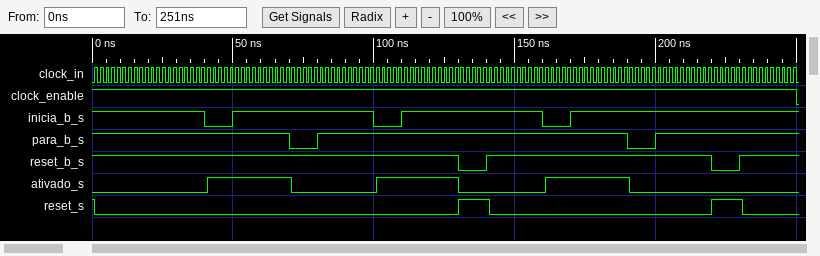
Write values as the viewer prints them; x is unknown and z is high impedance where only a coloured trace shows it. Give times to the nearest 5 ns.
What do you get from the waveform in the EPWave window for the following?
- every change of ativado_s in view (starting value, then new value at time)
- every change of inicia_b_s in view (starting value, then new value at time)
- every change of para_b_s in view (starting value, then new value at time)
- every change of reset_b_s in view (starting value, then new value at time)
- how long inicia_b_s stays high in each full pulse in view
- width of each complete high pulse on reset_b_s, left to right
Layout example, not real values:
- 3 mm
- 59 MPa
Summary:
- 0, 1 at 40 ns, 0 at 70 ns, 1 at 100 ns, 0 at 130 ns, 1 at 160 ns, 0 at 190 ns
- 1, 0 at 40 ns, 1 at 50 ns, 0 at 100 ns, 1 at 110 ns, 0 at 160 ns, 1 at 170 ns
- 1, 0 at 70 ns, 1 at 80 ns, 0 at 190 ns, 1 at 200 ns
- 1, 0 at 130 ns, 1 at 140 ns, 0 at 220 ns, 1 at 230 ns
- 50 ns, 50 ns
- 80 ns
